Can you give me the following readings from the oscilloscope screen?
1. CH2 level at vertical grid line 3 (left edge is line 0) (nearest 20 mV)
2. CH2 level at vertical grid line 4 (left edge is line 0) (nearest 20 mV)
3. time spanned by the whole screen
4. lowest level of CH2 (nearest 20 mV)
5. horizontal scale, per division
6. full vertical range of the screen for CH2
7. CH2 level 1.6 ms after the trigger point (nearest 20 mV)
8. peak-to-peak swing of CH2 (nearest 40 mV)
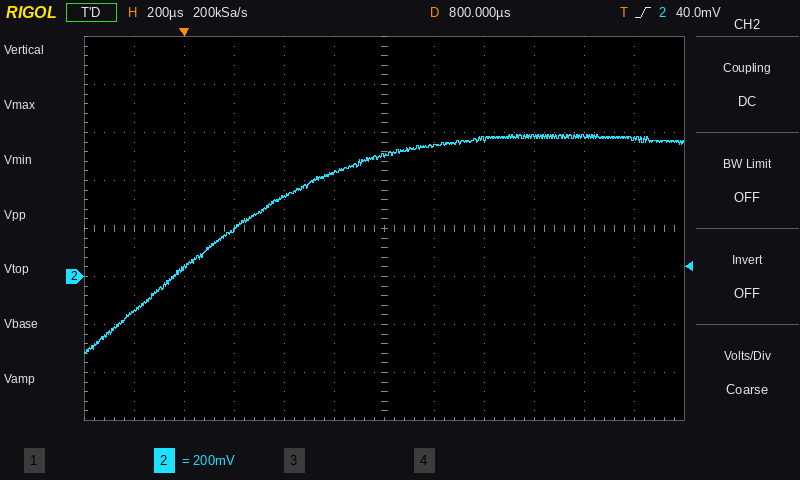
200 mV
340 mV
2.4 ms
-320 mV
200 µs
1.6 V
580 mV
920 mV
